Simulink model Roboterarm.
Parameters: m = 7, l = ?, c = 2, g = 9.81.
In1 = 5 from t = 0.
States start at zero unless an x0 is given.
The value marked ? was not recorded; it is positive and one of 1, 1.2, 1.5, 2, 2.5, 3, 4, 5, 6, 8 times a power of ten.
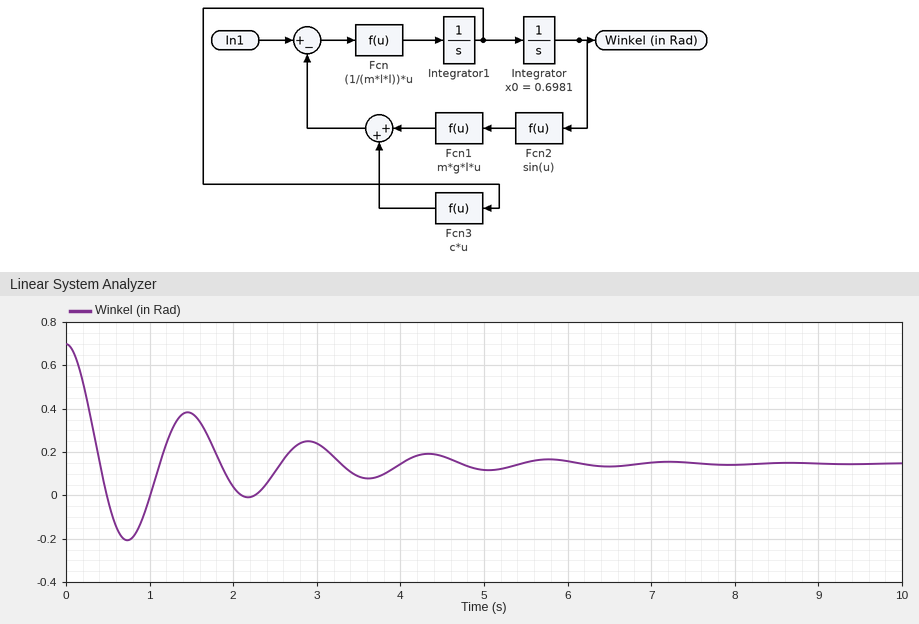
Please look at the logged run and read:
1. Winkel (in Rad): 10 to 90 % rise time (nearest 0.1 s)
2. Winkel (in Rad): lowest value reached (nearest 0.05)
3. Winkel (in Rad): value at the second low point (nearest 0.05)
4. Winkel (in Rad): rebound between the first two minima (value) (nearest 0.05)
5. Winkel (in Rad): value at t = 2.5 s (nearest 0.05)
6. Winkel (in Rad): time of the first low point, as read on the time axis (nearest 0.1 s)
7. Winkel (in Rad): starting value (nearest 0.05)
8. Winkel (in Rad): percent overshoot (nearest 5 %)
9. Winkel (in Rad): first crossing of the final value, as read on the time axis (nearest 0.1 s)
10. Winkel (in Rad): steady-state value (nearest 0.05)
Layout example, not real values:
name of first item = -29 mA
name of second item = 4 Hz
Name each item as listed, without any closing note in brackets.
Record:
Winkel (in Rad): 10 to 90 % rise time = 0.3 s
Winkel (in Rad): lowest value reached = -0.20
Winkel (in Rad): value at the second low point = 0.00
Winkel (in Rad): rebound between the first two minima (value) = 0.40
Winkel (in Rad): value at t = 2.5 s = 0.10
Winkel (in Rad): time of the first low point, as read on the time axis = 0.7 s
Winkel (in Rad): starting value = 0.70
Winkel (in Rad): percent overshoot = 65 %
Winkel (in Rad): first crossing of the final value, as read on the time axis = 0.4 s
Winkel (in Rad): steady-state value = 0.15
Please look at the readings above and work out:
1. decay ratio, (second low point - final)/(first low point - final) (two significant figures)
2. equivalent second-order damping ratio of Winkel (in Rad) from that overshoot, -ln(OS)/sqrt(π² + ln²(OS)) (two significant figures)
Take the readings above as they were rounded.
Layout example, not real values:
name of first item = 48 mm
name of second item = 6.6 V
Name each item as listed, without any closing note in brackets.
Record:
decay ratio, (second low point - final)/(first low point - final) = 0.43
equivalent second-order damping ratio of Winkel (in Rad) from that overshoot, -ln(OS)/sqrt(π² + ln²(OS)) = 0.14
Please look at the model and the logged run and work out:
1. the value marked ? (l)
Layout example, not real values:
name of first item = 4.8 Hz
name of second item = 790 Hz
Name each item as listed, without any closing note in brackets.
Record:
the value marked ? = 0.5
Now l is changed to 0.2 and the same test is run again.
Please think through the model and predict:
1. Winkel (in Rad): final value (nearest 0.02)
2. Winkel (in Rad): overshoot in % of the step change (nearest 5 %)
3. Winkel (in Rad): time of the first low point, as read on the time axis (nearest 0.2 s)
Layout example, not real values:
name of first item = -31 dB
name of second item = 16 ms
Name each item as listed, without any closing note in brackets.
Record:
Winkel (in Rad): final value = 0.38
Winkel (in Rad): overshoot in % of the step change = 15 %
Winkel (in Rad): time of the first low point, as read on the time axis = 0.6 s
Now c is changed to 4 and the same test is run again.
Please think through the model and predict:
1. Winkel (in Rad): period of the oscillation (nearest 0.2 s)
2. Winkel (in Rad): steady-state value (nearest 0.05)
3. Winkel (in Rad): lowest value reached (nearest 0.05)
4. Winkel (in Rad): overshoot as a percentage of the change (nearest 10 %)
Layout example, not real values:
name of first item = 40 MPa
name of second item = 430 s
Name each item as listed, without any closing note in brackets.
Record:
Winkel (in Rad): period of the oscillation = 1.4 s
Winkel (in Rad): steady-state value = 0.15
Winkel (in Rad): lowest value reached = -0.10
Winkel (in Rad): overshoot as a percentage of the change = 40 %
